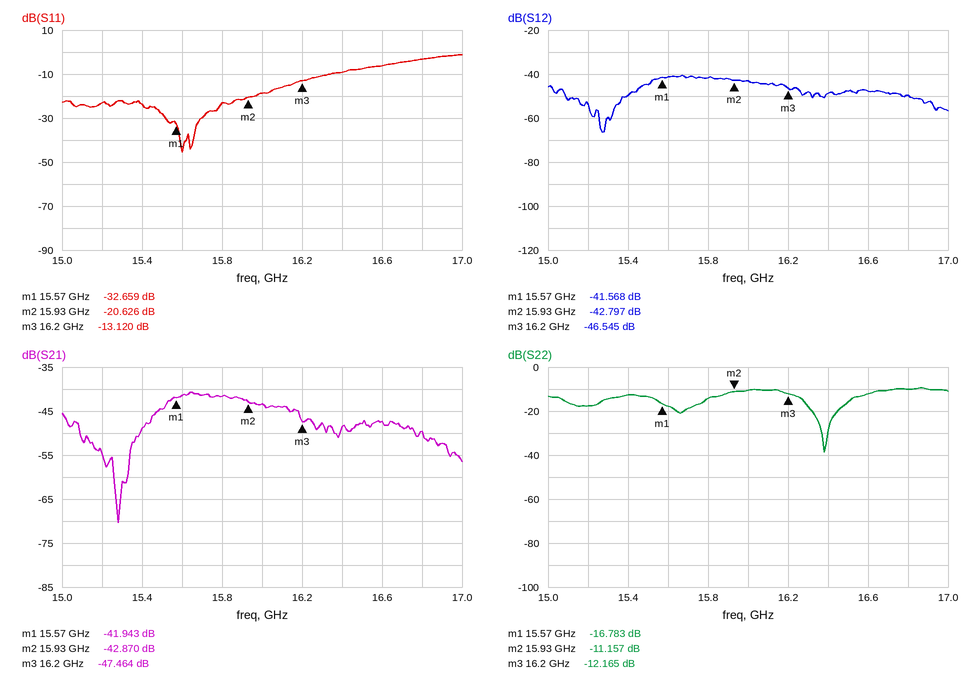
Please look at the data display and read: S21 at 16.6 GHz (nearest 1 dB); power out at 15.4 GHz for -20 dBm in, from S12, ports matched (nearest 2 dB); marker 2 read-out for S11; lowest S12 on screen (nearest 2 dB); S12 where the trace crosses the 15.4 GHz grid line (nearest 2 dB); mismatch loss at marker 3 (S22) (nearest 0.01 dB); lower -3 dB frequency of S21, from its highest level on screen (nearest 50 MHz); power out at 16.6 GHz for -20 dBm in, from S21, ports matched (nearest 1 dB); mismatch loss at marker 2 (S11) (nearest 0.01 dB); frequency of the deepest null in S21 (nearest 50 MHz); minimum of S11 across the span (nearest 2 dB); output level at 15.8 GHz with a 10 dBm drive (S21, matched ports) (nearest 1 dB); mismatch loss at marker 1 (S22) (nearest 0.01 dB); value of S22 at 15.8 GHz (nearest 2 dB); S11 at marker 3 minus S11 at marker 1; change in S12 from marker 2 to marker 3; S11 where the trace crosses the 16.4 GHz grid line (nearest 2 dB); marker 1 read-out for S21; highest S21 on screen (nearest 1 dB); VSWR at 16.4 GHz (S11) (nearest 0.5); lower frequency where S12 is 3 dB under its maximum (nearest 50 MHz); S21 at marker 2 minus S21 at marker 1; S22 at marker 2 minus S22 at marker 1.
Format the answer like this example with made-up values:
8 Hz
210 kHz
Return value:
-47 dB
-70 dBm
-20.626 dB
-66 dB
-50 dB
0.27 dB
15.50 GHz
-67 dBm
0.04 dB
15.30 GHz
-46 dB
-32 dBm
0.09 dB
-14 dB
19.539 dB
-3.748 dB
-10 dB
-41.943 dB
-41 dB
2.0
15.50 GHz
-0.927 dB
5.626 dB
